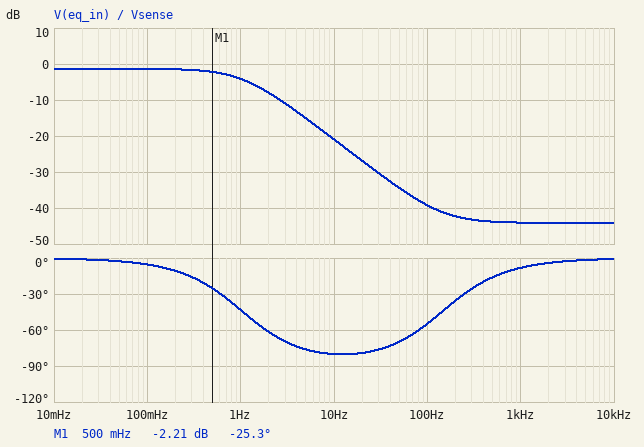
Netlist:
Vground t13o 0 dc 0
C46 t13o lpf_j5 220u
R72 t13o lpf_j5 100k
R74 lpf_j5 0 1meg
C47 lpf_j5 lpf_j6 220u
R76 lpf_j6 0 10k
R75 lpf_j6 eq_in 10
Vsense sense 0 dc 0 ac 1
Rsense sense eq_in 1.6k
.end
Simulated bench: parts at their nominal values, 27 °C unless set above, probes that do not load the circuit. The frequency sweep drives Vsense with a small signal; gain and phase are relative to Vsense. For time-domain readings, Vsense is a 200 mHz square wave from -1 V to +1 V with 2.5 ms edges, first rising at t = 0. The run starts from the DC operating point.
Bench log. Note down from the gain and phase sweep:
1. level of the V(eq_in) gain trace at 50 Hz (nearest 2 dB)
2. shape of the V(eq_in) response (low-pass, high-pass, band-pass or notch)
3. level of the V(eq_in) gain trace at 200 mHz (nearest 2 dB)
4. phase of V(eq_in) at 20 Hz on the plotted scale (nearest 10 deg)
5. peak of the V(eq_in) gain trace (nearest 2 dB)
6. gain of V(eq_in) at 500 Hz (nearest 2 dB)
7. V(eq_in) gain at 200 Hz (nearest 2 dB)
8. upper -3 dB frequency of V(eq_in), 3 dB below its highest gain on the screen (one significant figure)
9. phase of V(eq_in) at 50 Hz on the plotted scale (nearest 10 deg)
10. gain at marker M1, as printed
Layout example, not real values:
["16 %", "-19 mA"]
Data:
["-34 dB", "low-pass", "-2 dB", "-80 deg", "-2 dB", "-44 dB", "-42 dB", "1 Hz", "-70 deg", "-2.21 dB"]
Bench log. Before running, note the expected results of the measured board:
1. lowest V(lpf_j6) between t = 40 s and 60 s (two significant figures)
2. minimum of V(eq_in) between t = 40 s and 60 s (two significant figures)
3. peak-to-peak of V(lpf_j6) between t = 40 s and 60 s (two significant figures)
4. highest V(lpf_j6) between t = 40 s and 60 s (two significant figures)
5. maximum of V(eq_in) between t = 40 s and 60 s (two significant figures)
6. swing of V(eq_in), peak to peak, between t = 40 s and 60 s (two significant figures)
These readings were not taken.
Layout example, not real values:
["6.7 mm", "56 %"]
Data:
["-860 mV", "-860 mV", "1.7 V", "860 mV", "860 mV", "1.7 V"]
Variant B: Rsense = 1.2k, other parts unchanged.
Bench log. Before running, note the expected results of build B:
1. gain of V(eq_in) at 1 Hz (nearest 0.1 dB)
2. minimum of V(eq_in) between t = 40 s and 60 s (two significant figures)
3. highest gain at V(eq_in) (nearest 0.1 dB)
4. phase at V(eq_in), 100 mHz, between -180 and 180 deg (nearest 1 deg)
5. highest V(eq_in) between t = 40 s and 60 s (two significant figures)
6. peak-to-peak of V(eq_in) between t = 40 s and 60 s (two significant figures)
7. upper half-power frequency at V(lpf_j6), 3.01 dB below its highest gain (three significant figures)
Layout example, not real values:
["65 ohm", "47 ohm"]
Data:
["-2.9 dB", "-890 mV", "-1.0 dB", "-4 deg", "890 mV", "1.8 V", "1.34 Hz"]
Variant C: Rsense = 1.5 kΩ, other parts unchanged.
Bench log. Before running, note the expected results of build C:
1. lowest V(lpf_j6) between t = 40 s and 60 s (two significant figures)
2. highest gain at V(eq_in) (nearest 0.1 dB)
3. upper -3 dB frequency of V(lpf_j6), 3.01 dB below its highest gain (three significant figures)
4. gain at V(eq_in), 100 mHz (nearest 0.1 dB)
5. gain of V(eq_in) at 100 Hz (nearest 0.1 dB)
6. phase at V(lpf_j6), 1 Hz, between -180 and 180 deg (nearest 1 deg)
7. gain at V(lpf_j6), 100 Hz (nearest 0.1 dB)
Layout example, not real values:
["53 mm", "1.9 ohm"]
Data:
["-870 mV", "-1.2 dB", "1.10 Hz", "-1.3 dB", "-38.7 dB", "-42 deg", "-40.4 dB"]
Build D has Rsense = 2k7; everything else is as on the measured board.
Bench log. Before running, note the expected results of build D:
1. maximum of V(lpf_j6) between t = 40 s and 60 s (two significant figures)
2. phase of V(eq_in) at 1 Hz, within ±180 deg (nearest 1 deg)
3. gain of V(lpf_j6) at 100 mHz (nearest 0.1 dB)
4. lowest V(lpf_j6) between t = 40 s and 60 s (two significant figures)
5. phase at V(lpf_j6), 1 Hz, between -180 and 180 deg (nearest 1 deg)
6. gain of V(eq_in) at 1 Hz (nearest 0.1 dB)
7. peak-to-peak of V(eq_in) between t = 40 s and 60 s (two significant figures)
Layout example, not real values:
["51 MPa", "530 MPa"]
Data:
["780 mV", "-55 deg", "-2.2 dB", "-780 mV", "-56 deg", "-7.1 dB", "1.6 V"]
